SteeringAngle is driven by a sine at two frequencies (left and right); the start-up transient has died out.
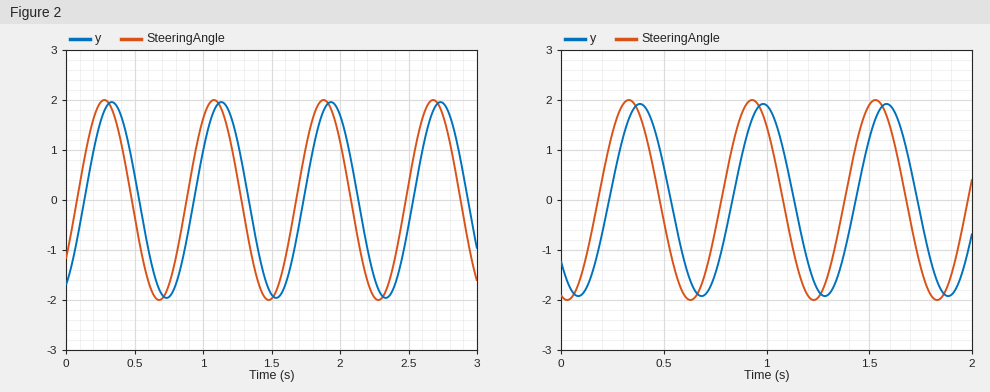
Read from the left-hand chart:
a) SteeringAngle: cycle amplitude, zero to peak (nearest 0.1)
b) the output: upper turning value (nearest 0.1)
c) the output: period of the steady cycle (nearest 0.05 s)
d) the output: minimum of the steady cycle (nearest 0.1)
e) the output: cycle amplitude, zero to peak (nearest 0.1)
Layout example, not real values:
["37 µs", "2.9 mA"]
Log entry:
["2.0", "2.0", "0.80 s", "-2.0", "2.0"]
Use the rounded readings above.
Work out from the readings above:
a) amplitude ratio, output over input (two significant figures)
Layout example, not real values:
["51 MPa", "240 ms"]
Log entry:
["1.0"]
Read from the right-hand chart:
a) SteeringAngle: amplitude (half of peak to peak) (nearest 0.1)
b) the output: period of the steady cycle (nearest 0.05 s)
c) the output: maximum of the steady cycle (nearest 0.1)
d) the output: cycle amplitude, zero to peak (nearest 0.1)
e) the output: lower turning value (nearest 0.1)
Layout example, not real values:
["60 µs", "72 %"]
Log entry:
["2.0", "0.60 s", "1.9", "1.9", "-1.9"]
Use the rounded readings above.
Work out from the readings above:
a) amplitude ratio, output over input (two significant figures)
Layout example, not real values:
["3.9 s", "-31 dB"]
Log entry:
["0.95"]
